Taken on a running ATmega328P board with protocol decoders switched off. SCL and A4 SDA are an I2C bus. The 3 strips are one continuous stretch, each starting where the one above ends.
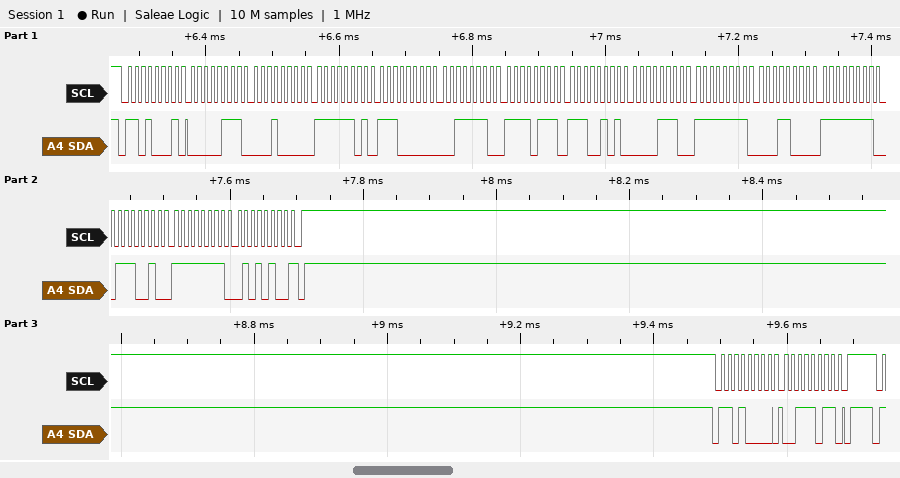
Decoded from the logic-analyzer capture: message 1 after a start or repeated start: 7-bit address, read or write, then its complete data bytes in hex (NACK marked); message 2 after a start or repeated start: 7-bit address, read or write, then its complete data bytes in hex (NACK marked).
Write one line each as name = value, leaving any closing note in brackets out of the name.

message 1 after a start or repeated start: 7-bit address, read or write, then its complete data bytes in hex = 0x68 read: 07 10 FD E0 3E F7 E5 0E FF 18 FF 72 FF 54 NACK
message 2 after a start or repeated start: 7-bit address, read or write, then its complete data bytes in hex = 0x68 write: 3B
